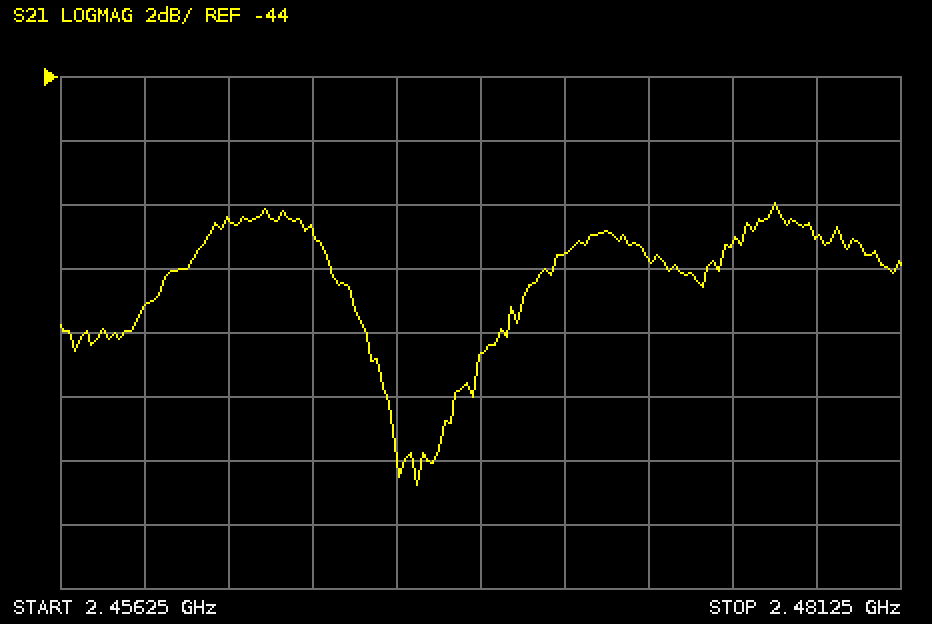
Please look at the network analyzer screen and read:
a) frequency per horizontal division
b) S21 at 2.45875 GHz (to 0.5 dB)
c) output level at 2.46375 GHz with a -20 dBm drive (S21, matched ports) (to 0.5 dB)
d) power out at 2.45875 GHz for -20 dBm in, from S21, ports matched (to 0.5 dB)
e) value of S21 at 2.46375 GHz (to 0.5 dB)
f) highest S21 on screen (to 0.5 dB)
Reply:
2.5 MHz
-51.0 dB
-69.0 dBm
-71.0 dBm
-49.0 dB
-48.0 dB
